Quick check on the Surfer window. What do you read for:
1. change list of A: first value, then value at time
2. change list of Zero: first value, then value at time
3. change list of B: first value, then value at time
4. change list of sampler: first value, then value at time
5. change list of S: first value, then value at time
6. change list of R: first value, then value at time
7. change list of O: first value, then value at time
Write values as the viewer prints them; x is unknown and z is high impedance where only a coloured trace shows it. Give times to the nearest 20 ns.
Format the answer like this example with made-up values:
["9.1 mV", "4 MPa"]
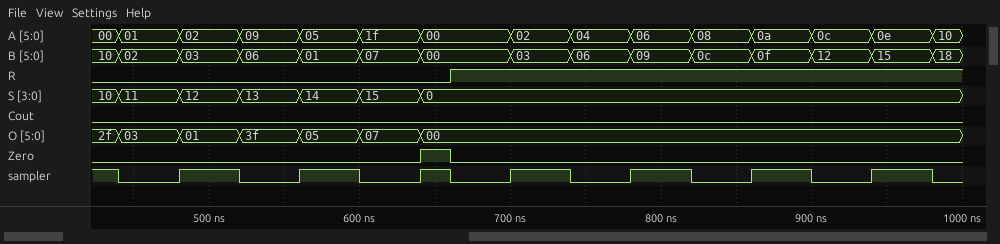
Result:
["00, 01 at 440 ns, 02 at 480 ns, 09 at 520 ns, 05 at 560 ns, 1f at 600 ns, 00 at 640 ns, 02 at 700 ns, 04 at 740 ns, 06 at 780 ns, 08 at 820 ns, 0a at 860 ns, 0c at 900 ns, 0e at 940 ns, 10 at 980 ns", "0, 1 at 640 ns, 0 at 660 ns", "10, 02 at 440 ns, 03 at 480 ns, 06 at 520 ns, 01 at 560 ns, 07 at 600 ns, 00 at 640 ns, 03 at 700 ns, 06 at 740 ns, 09 at 780 ns, 0c at 820 ns, 0f at 860 ns, 12 at 900 ns, 15 at 940 ns, 18 at 980 ns", "1, 0 at 440 ns, 1 at 480 ns, 0 at 520 ns, 1 at 560 ns, 0 at 600 ns, 1 at 640 ns, 0 at 660 ns, 1 at 700 ns, 0 at 740 ns, 1 at 780 ns, 0 at 820 ns, 1 at 860 ns, 0 at 900 ns, 1 at 940 ns, 0 at 980 ns", "10, 11 at 440 ns, 12 at 480 ns, 13 at 520 ns, 14 at 560 ns, 15 at 600 ns, 0 at 640 ns", "0, 1 at 660 ns", "2f, 03 at 440 ns, 01 at 480 ns, 3f at 520 ns, 05 at 560 ns, 07 at 600 ns, 00 at 640 ns"]
